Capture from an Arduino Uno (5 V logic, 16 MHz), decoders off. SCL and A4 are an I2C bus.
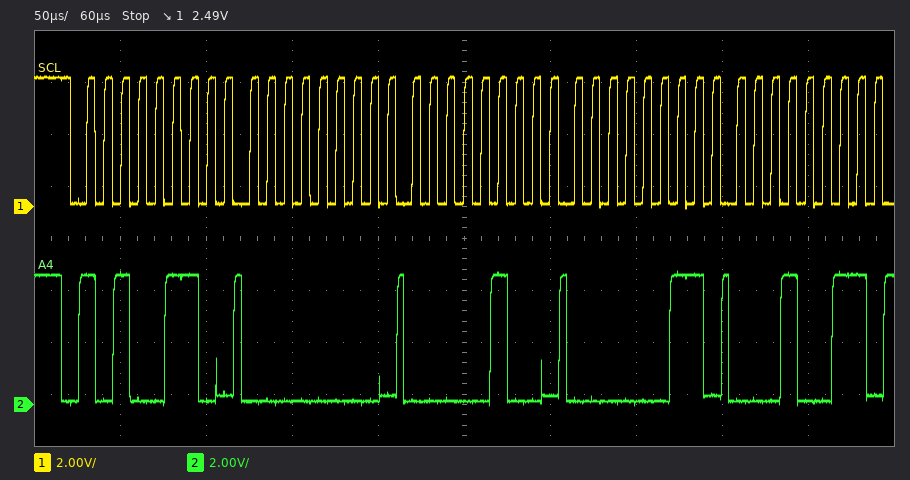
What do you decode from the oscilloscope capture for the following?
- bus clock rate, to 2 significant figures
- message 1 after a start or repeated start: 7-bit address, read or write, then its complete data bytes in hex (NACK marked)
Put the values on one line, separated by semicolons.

100 kHz; 0x53 write: 00 04 03 13
